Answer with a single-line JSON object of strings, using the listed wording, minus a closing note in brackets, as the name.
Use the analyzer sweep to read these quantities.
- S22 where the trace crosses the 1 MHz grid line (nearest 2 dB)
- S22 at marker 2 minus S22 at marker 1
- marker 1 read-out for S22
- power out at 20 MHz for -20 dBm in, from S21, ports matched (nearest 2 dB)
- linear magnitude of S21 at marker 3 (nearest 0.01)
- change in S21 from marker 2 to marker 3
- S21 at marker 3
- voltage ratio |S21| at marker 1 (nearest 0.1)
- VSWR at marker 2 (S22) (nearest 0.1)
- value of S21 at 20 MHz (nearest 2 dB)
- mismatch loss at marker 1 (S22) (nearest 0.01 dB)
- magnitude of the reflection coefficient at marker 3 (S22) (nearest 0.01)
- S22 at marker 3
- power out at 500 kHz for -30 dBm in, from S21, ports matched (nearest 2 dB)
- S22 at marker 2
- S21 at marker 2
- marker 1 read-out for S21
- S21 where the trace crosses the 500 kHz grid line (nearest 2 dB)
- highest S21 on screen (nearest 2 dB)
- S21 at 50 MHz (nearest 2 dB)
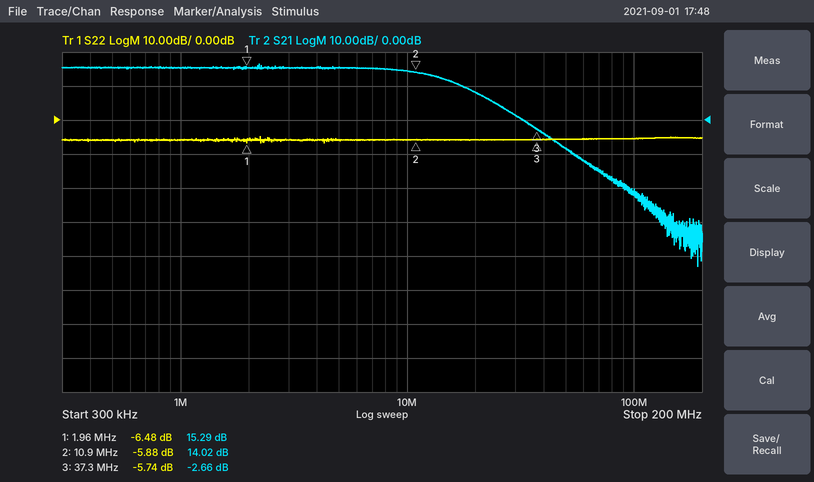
{"S22 where the trace crosses the 1 MHz grid line": "-6 dB", "S22 at marker 2 minus S22 at marker 1": "0.60 dB", "marker 1 read-out for S22": "-6.48 dB", "power out at 20 MHz for -20 dBm in, from S21, ports matched": "-12 dBm", "linear magnitude of S21 at marker 3": "0.74", "change in S21 from marker 2 to marker 3": "-16.68 dB", "S21 at marker 3": "-2.66 dB", "voltage ratio |S21| at marker 1": "5.8", "VSWR at marker 2 (S22)": "3.1", "value of S21 at 20 MHz": "8 dB", "mismatch loss at marker 1 (S22)": "1.11 dB", "magnitude of the reflection coefficient at marker 3 (S22)": "0.52", "S22 at marker 3": "-5.74 dB", "power out at 500 kHz for -30 dBm in, from S21, ports matched": "-14 dBm", "S22 at marker 2": "-5.88 dB", "S21 at marker 2": "14.02 dB", "marker 1 read-out for S21": "15.29 dB", "S21 where the trace crosses the 500 kHz grid line": "16 dB", "highest S21 on screen": "16 dB", "S21 at 50 MHz": "-8 dB"}
